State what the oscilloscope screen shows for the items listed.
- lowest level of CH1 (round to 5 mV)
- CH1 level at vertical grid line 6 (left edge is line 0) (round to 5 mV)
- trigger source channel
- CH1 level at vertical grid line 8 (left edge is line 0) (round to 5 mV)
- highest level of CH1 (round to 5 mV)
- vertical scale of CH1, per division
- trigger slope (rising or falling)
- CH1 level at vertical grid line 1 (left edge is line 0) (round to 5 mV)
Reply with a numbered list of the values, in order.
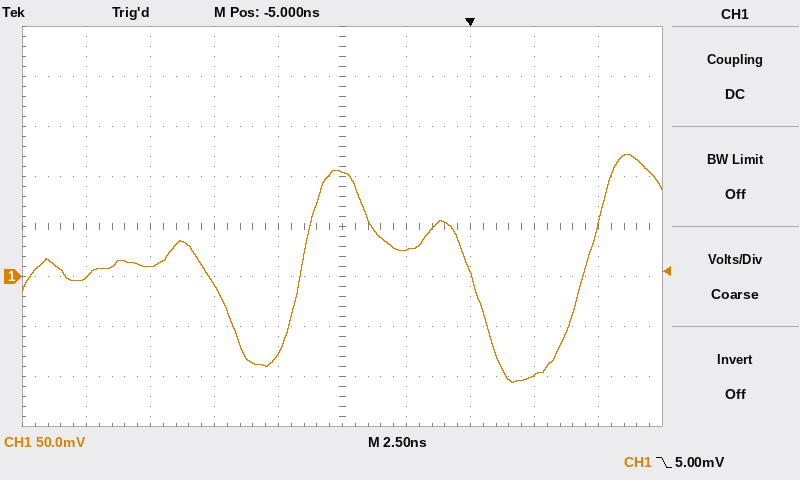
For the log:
1. -105 mV
2. 25 mV
3. CH1
4. -100 mV
5. 120 mV
6. 50 mV
7. falling
8. 0 mV
